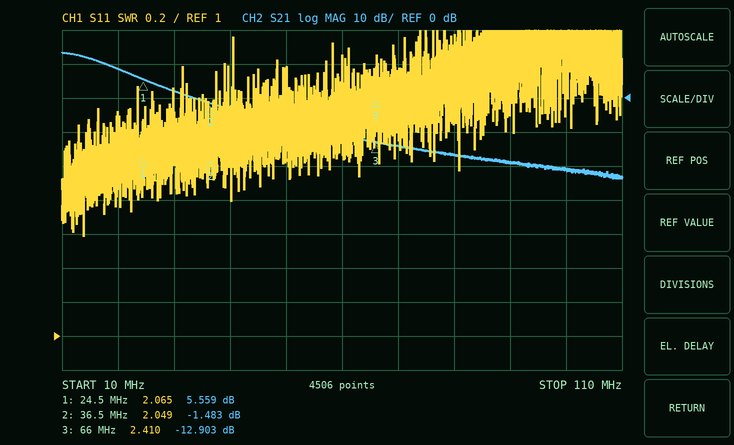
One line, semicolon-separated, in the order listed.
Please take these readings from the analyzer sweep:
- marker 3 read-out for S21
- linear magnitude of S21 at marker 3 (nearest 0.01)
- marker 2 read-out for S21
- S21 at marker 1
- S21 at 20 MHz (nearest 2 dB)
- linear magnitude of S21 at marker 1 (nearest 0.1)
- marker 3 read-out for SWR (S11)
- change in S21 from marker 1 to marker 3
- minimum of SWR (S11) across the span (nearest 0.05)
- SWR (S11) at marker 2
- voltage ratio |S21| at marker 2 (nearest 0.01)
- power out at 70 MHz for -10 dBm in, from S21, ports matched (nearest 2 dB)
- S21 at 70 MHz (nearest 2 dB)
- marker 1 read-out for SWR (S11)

-12.903 dB; 0.23; -1.483 dB; 5.559 dB; 8 dB; 1.9; 2.410; -18.462 dB; 1.60; 2.049; 0.84; -24 dBm; -14 dB; 2.065
